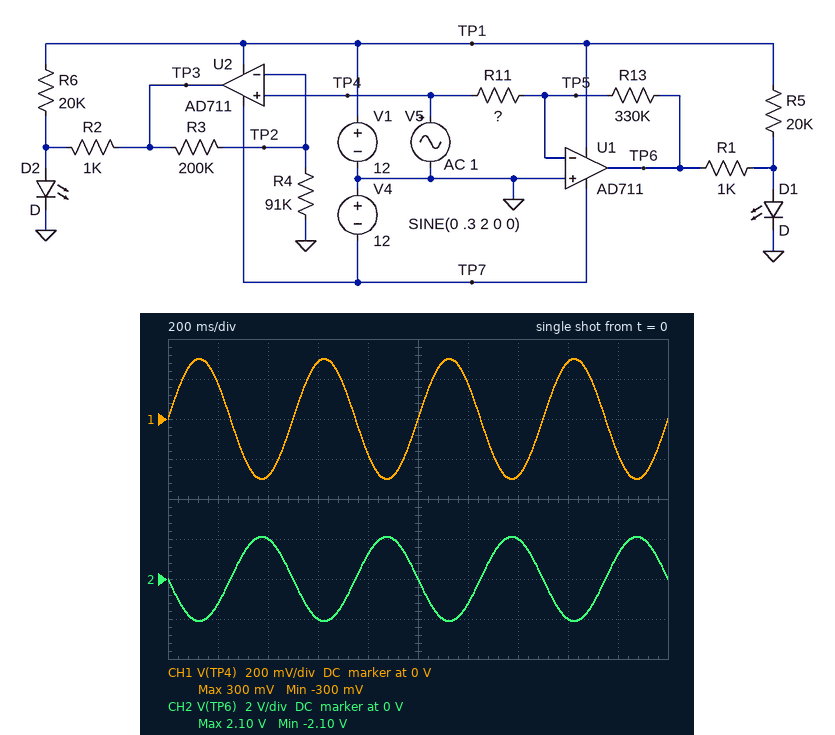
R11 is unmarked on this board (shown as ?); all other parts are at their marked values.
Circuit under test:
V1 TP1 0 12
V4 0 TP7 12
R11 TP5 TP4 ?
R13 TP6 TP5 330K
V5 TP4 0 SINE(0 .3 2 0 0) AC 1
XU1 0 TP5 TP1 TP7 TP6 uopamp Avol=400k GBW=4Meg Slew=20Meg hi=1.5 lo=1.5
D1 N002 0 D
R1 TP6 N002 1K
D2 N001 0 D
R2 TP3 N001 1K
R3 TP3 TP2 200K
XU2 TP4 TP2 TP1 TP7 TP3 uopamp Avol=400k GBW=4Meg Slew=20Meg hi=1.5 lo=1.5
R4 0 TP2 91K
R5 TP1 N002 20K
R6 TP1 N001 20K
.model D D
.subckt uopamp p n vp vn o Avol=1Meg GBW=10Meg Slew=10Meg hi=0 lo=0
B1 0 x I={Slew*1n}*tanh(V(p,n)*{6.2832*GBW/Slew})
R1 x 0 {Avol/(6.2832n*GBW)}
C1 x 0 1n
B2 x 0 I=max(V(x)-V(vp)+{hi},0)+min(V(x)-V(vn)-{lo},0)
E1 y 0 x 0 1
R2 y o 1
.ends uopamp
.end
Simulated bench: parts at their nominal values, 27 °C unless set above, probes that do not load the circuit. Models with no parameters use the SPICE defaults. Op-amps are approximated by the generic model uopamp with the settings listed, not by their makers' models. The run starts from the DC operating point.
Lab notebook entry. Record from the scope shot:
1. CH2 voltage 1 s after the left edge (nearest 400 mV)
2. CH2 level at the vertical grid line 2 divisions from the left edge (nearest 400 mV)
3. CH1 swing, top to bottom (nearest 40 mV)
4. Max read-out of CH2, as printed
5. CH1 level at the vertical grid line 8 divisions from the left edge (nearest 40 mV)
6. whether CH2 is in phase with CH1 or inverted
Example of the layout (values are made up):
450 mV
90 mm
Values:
0 V
2.0 V
600 mV
2.10 V
280 mV
inverted
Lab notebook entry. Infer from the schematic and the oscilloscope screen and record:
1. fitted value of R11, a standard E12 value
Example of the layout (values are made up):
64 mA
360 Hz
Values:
47 kΩ
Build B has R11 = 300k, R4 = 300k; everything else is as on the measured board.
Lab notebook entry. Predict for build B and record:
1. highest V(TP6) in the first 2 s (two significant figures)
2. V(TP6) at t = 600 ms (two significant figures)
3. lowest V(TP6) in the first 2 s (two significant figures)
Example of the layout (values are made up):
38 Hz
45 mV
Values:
330 mV
-310 mV
-330 mV
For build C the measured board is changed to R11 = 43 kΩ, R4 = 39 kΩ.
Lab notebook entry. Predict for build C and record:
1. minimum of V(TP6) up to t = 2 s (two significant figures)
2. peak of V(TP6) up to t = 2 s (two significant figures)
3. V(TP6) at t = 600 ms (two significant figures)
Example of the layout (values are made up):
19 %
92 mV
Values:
-2.3 V
2.3 V
-2.2 V
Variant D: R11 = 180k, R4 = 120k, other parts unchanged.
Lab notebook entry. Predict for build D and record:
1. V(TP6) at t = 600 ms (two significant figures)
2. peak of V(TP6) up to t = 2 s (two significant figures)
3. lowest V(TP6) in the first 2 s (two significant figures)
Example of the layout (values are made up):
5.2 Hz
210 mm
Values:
-520 mV
550 mV
-550 mV
